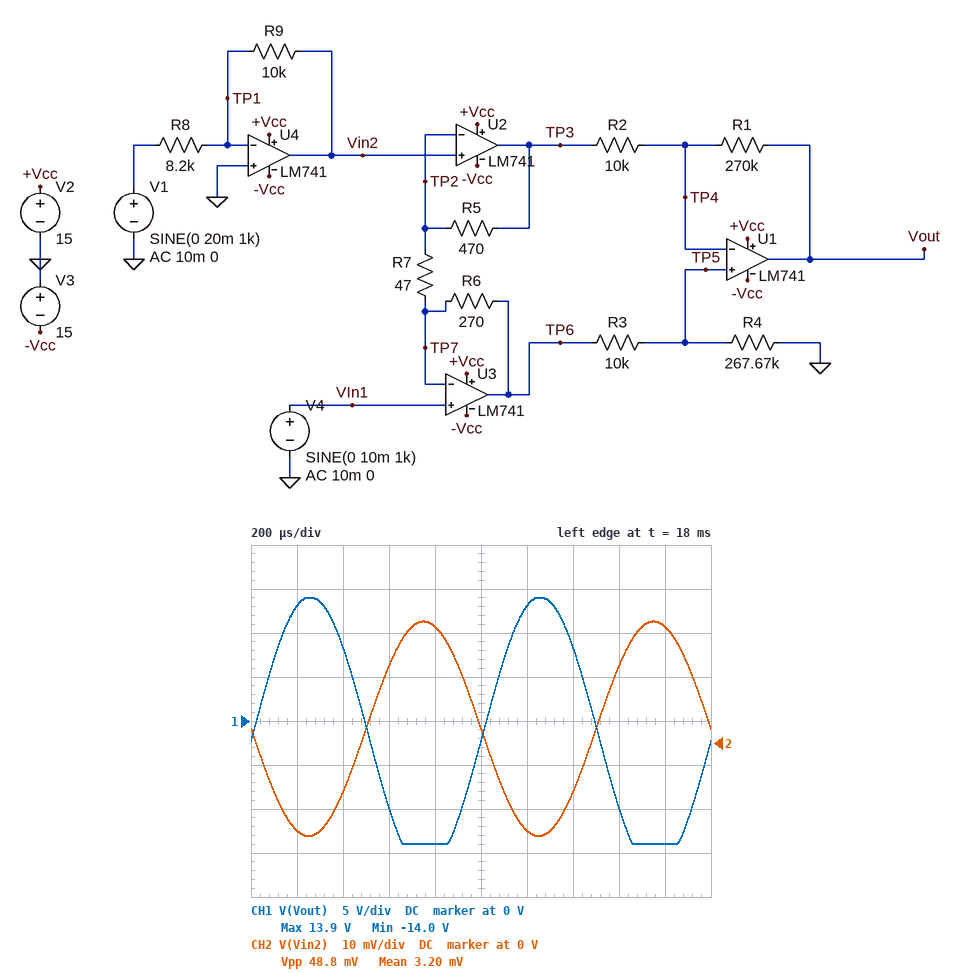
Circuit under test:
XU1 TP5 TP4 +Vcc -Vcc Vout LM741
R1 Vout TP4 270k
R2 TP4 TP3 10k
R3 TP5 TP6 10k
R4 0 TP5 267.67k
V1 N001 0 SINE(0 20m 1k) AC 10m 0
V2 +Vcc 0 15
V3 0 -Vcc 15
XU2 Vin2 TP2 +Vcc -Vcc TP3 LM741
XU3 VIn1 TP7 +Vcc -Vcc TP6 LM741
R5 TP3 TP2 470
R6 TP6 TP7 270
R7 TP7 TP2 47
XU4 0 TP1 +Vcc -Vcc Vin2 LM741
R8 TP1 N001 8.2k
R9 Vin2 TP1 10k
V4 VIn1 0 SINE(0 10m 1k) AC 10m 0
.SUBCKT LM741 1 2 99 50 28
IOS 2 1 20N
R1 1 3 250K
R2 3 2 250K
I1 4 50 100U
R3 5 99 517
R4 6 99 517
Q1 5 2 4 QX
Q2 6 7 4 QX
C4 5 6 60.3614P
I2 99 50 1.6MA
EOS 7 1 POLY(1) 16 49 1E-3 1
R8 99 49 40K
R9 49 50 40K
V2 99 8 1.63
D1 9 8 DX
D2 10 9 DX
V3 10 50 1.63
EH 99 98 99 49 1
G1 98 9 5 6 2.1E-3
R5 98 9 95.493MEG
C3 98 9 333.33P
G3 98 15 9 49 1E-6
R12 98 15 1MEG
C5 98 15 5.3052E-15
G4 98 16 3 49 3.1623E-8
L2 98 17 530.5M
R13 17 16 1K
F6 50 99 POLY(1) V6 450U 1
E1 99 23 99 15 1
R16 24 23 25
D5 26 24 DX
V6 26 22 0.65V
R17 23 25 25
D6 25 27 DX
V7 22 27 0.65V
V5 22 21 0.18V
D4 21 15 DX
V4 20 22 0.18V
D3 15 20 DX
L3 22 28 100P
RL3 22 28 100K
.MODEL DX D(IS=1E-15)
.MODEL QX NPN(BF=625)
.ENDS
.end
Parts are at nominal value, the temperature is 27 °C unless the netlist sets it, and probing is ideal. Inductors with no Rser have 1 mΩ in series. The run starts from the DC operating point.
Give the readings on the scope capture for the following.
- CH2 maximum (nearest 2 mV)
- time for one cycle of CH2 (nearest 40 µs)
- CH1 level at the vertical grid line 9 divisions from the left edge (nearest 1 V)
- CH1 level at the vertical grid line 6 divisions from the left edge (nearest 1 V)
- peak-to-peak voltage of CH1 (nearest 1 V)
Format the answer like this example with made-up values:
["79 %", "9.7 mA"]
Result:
["28 mV", "1.00 ms", "-14 V", "13 V", "28 V"]
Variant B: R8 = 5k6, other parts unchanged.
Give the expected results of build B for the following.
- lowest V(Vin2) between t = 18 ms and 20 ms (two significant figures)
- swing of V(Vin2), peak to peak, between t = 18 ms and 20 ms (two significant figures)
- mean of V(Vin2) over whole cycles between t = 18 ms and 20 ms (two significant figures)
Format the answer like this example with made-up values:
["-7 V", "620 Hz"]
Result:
["-32 mV", "71 mV", "3.8 mV"]
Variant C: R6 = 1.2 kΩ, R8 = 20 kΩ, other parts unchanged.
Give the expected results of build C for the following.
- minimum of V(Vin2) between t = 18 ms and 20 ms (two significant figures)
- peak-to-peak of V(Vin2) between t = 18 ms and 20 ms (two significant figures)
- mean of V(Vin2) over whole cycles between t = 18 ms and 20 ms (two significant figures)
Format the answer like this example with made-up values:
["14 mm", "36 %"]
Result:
["-7.5 mV", "20 mV", "2.5 mV"]
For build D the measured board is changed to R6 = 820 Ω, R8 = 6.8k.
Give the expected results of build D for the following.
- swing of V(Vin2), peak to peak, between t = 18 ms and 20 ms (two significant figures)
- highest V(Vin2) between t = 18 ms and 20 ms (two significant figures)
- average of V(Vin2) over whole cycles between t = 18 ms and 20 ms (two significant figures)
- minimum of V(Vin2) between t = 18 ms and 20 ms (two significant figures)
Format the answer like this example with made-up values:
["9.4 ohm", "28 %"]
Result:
["59 mV", "33 mV", "3.5 mV", "-26 mV"]
